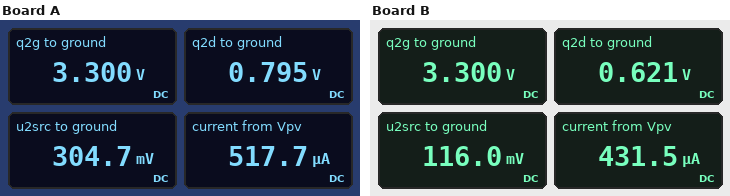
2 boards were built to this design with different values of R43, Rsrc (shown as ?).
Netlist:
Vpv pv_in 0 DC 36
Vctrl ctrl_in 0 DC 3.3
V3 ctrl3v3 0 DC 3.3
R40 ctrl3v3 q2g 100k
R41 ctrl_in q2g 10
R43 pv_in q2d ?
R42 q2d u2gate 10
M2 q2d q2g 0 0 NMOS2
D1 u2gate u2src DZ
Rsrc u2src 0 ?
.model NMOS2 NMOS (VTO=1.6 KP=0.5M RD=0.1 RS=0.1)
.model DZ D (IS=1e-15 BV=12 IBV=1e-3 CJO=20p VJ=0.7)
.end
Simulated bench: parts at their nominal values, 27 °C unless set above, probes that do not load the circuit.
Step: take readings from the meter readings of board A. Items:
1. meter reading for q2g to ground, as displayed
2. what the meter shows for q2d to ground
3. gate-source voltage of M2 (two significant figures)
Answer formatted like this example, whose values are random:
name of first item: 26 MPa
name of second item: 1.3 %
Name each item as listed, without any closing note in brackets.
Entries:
meter reading for q2g to ground, as displayed: 3.300 V
what the meter shows for q2d to ground: 0.795 V
gate-source voltage of M2: 3.3 V
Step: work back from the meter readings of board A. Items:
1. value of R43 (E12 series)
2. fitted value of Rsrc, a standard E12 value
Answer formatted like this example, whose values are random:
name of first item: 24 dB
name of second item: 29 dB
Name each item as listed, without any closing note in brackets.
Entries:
value of R43: 68 kΩ
fitted value of Rsrc, a standard E12 value: 1.8 MΩ
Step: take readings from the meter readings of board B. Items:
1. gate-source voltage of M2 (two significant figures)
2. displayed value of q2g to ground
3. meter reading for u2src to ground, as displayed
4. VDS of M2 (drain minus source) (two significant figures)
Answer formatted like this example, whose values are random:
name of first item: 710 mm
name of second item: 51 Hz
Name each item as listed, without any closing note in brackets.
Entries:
gate-source voltage of M2: 3.3 V
displayed value of q2g to ground: 3.300 V
meter reading for u2src to ground, as displayed: 116.0 mV
VDS of M2 (drain minus source): 620 mV
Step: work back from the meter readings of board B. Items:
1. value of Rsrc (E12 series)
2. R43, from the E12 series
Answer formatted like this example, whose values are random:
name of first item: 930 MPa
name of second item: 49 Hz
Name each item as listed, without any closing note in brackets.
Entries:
value of Rsrc: 390 kΩ
R43, from the E12 series: 82 kΩ
